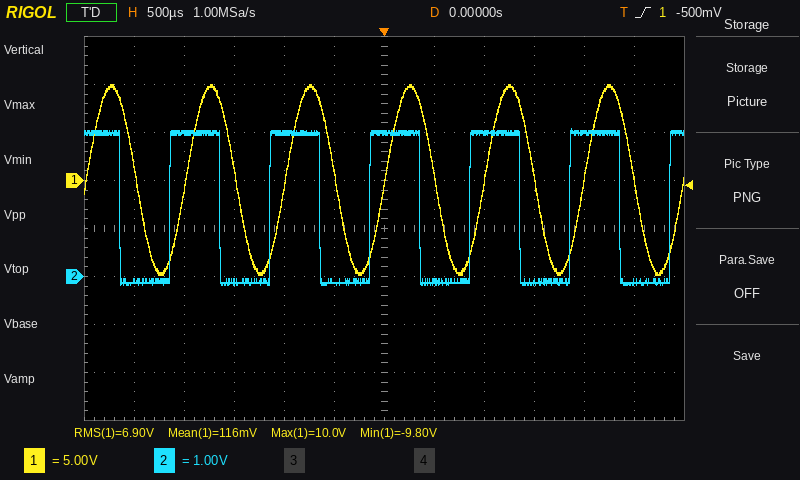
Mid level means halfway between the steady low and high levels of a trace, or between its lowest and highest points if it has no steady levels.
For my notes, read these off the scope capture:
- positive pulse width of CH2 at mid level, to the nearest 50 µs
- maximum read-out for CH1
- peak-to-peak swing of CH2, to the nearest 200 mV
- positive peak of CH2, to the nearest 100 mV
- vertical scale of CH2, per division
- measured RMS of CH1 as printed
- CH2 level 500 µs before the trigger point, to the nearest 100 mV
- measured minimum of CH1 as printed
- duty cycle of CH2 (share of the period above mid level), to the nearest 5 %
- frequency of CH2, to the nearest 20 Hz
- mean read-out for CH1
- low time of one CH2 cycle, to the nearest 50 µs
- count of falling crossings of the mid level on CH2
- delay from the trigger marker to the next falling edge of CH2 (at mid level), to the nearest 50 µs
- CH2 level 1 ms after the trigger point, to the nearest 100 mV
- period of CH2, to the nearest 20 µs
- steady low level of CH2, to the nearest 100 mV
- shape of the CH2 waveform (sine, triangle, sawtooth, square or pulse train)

500 µs
10.0 V
3.2 V
3.1 V
1 V
6.90 V
-100 mV
-9.80 V
50 %
1.00 kHz
116 mV
500 µs
6
350 µs
3.0 V
1.00 ms
-100 mV
square
